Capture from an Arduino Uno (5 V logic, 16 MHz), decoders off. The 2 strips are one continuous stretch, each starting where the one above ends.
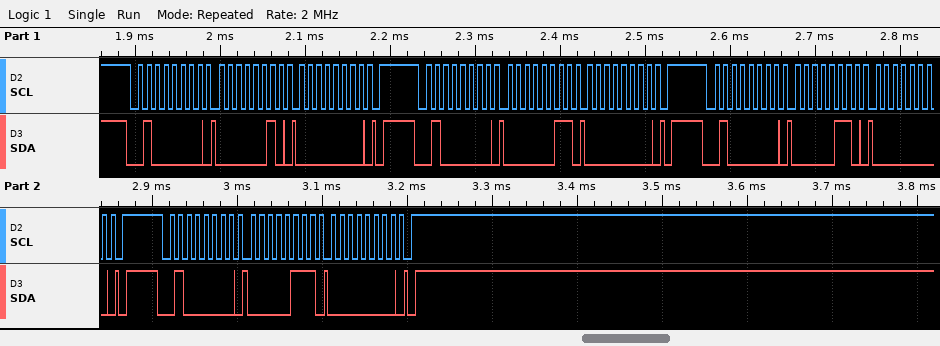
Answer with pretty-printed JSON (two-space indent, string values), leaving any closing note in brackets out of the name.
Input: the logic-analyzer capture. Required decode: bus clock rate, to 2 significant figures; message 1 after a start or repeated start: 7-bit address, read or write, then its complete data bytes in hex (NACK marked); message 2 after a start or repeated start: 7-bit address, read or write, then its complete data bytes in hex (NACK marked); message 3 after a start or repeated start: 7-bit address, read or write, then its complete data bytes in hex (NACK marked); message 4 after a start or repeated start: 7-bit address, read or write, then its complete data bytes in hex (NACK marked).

{
  "bus clock rate, to 2 significant figures": "100 kHz",
  "message 1 after a start or repeated start: 7-bit address, read or write, then its complete data bytes in hex": "0x20 write: 02 00",
  "message 2 after a start or repeated start: 7-bit address, read or write, then its complete data bytes in hex": "0x20 write: 03 00",
  "message 3 after a start or repeated start: 7-bit address, read or write, then its complete data bytes in hex": "0x20 write: 06 00",
  "message 4 after a start or repeated start: 7-bit address, read or write, then its complete data bytes in hex": "0x20 write: 07 00"
}
